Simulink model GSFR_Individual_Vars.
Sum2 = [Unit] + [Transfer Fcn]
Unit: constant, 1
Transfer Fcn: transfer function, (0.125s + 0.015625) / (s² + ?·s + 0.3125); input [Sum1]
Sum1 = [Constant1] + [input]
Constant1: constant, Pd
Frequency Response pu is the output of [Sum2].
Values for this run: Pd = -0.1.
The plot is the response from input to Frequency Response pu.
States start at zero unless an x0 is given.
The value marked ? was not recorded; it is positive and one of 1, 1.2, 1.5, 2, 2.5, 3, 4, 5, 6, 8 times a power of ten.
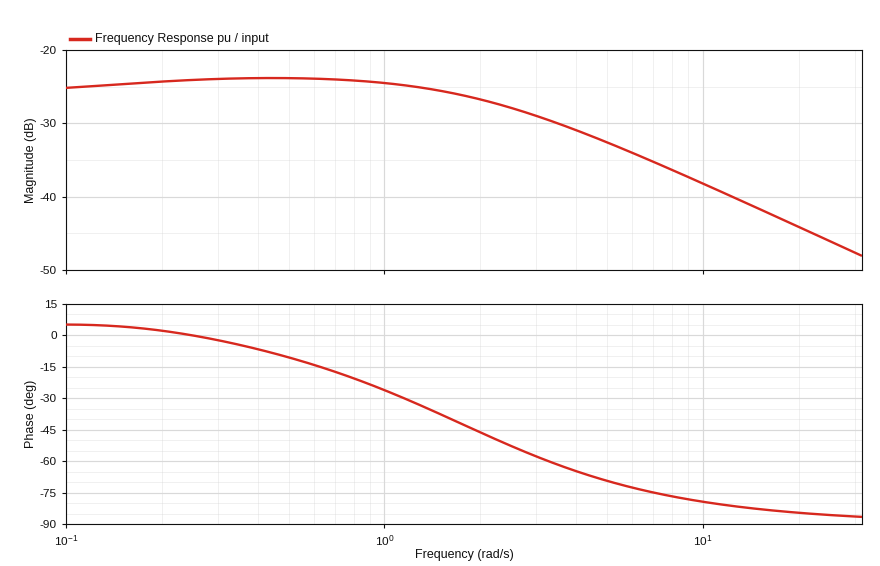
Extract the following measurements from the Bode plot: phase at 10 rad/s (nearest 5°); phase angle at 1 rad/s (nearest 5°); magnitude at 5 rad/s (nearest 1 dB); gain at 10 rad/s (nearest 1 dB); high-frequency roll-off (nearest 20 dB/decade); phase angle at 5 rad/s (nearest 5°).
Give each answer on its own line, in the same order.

-80°
-25°
-33 dB
-38 dB
-20 dB/decade
-70°
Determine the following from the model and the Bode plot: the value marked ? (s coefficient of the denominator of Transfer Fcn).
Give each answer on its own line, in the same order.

2
